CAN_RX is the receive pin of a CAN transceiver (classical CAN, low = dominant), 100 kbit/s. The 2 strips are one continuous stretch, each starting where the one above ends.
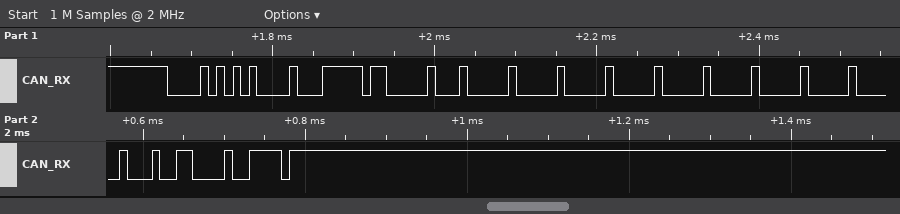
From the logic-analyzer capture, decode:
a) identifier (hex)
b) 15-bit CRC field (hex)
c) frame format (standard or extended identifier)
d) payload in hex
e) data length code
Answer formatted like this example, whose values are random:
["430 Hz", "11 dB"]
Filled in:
["0x0AA", "0x4C27", "standard", "FE 01 00 00 00 00 00 00", "8"]
